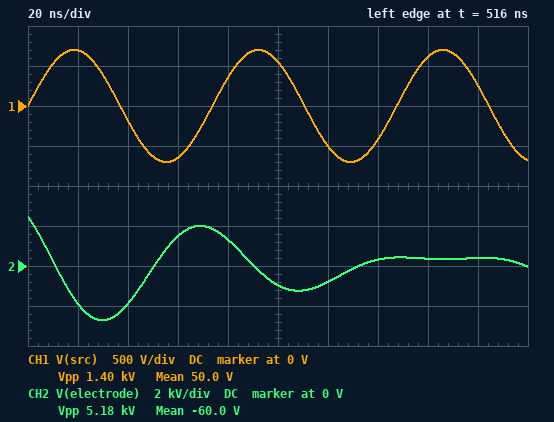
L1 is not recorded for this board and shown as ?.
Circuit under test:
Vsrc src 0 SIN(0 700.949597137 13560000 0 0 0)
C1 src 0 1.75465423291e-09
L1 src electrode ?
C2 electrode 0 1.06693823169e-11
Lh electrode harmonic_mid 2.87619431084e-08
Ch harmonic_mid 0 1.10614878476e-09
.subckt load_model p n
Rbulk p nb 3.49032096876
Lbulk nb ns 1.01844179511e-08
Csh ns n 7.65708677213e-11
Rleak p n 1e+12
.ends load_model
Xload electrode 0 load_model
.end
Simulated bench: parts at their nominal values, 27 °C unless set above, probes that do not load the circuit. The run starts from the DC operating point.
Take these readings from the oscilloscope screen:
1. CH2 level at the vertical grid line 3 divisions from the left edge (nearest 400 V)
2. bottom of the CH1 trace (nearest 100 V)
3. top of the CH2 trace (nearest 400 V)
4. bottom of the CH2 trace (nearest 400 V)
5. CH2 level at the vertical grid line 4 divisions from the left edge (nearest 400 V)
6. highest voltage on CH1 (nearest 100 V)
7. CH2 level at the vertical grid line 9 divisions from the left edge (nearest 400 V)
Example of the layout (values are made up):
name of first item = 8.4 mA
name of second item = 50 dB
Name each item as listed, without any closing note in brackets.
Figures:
CH2 level at the vertical grid line 3 divisions from the left edge = 1.6 kV
bottom of the CH1 trace = -700 V
top of the CH2 trace = 2.4 kV
bottom of the CH2 trace = -2.8 kV
CH2 level at the vertical grid line 4 divisions from the left edge = 1.2 kV
highest voltage on CH1 = 700 V
CH2 level at the vertical grid line 9 divisions from the left edge = 400 V
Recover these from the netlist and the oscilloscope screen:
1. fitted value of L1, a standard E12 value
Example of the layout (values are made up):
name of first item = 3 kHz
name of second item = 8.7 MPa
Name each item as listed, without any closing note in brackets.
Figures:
fitted value of L1, a standard E12 value = 120 nH
